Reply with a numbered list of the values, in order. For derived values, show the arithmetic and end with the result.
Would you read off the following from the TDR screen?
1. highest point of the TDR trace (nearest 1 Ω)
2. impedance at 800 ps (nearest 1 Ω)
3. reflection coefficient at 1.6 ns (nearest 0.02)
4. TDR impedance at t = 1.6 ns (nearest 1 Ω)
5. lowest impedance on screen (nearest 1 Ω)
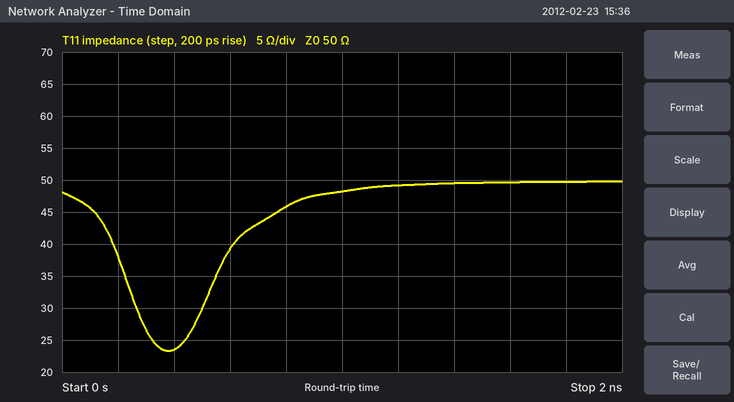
1. 50 Ω
2. 46 Ω
3. (50 − 50)/(50 + 50) ≈ 0.00
4. 50 Ω
5. 23 Ω
